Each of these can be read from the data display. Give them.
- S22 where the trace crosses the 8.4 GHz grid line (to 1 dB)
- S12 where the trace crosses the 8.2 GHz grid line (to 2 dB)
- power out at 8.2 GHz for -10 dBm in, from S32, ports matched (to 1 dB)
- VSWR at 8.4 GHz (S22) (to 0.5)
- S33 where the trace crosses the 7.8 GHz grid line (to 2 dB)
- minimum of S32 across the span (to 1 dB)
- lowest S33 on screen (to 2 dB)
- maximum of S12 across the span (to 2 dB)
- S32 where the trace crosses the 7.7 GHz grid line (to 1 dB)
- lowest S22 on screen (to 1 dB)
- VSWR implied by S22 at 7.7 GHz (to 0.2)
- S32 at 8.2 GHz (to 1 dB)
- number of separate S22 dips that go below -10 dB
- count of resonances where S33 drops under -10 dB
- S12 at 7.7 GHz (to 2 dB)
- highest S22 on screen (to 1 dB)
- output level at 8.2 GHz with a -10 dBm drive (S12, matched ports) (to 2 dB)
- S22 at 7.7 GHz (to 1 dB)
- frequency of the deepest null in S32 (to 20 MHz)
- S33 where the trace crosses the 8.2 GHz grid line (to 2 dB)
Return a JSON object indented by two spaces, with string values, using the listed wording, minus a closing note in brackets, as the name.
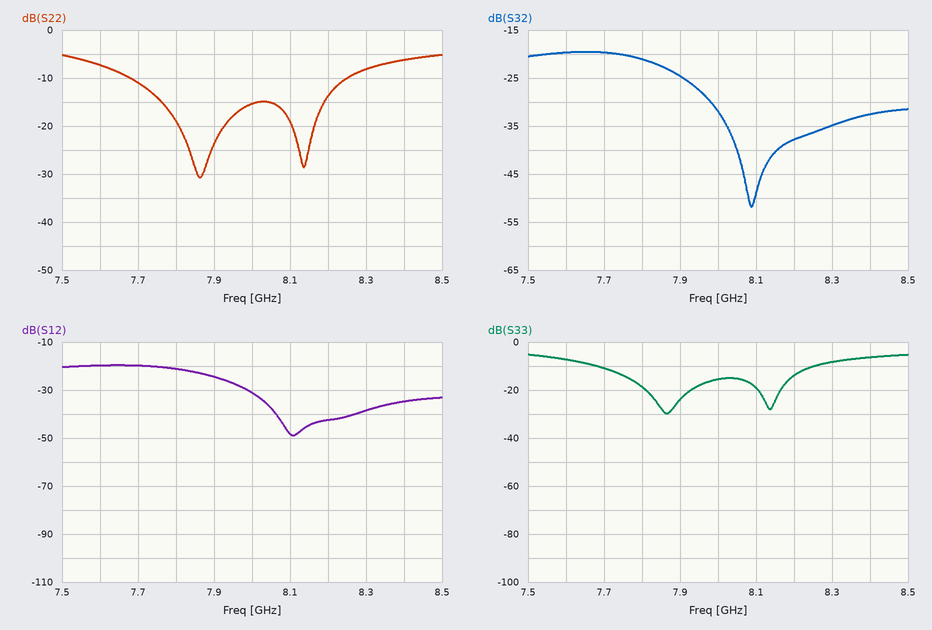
{
  "S22 where the trace crosses the 8.4 GHz grid line": "-6 dB",
  "S12 where the trace crosses the 8.2 GHz grid line": "-42 dB",
  "power out at 8.2 GHz for -10 dBm in, from S32, ports matched": "-48 dBm",
  "VSWR at 8.4 GHz (S22)": "3.0",
  "S33 where the trace crosses the 7.8 GHz grid line": "-18 dB",
  "minimum of S32 across the span": "-52 dB",
  "lowest S33 on screen": "-30 dB",
  "maximum of S12 across the span": "-20 dB",
  "S32 where the trace crosses the 7.7 GHz grid line": "-20 dB",
  "lowest S22 on screen": "-31 dB",
  "VSWR implied by S22 at 7.7 GHz": "1.8",
  "S32 at 8.2 GHz": "-38 dB",
  "number of separate S22 dips that go below -10 dB": "2",
  "count of resonances where S33 drops under -10 dB": "2",
  "S12 at 7.7 GHz": "-20 dB",
  "highest S22 on screen": "-5 dB",
  "output level at 8.2 GHz with a -10 dBm drive (S12, matched ports)": "-52 dBm",
  "S22 at 7.7 GHz": "-11 dB",
  "frequency of the deepest null in S32": "8.08 GHz",
  "S33 where the trace crosses the 8.2 GHz grid line": "-14 dB"
}
